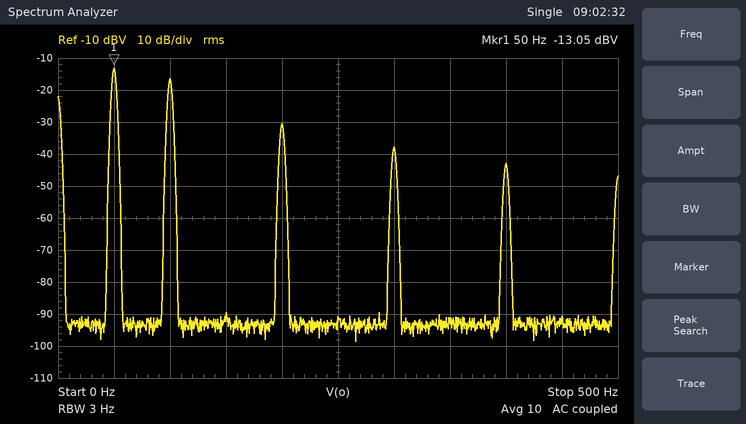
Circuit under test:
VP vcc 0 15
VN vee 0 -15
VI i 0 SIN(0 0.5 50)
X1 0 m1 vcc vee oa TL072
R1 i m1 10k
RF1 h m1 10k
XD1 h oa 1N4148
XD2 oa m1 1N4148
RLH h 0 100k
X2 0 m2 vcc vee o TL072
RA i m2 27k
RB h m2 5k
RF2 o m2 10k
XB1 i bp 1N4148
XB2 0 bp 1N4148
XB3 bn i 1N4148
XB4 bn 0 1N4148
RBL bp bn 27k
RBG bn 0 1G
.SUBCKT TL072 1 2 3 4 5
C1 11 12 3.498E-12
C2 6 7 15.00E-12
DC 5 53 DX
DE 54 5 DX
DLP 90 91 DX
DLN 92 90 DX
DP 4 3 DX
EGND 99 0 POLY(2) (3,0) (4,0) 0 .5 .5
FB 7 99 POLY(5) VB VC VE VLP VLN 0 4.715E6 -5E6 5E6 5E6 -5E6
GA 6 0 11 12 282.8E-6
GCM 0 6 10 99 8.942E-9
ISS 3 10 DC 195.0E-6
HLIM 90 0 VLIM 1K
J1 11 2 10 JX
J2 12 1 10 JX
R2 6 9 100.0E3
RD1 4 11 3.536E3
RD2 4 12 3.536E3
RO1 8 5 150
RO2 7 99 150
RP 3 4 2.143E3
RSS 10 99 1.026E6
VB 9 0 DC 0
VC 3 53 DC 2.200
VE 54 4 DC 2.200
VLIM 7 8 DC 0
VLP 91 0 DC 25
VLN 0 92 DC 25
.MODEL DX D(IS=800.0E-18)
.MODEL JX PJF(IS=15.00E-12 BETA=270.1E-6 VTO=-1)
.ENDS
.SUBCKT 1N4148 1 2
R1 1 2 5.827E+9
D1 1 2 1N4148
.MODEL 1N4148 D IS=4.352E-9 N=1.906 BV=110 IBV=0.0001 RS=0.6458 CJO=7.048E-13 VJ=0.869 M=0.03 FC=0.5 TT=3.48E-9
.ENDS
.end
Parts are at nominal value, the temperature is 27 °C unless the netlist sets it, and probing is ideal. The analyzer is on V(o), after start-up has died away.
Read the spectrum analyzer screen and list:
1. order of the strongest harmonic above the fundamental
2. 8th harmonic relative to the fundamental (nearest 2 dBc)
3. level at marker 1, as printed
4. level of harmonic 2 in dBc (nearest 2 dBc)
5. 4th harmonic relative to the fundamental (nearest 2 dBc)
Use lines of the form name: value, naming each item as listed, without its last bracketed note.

order of the strongest harmonic above the fundamental: 2
8th harmonic relative to the fundamental: -30 dBc
level at marker 1, as printed: -13.05 dBV
level of harmonic 2 in dBc: -4 dBc
4th harmonic relative to the fundamental: -18 dBc
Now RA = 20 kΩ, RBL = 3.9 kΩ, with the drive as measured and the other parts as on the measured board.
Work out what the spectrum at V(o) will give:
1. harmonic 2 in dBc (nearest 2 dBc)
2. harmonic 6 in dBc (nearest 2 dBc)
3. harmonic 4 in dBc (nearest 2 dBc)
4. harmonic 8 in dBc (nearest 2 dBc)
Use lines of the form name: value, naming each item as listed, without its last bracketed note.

harmonic 2 in dBc: -2 dBc
harmonic 6 in dBc: -22 dBc
harmonic 4 in dBc: -16 dBc
harmonic 8 in dBc: -28 dBc
